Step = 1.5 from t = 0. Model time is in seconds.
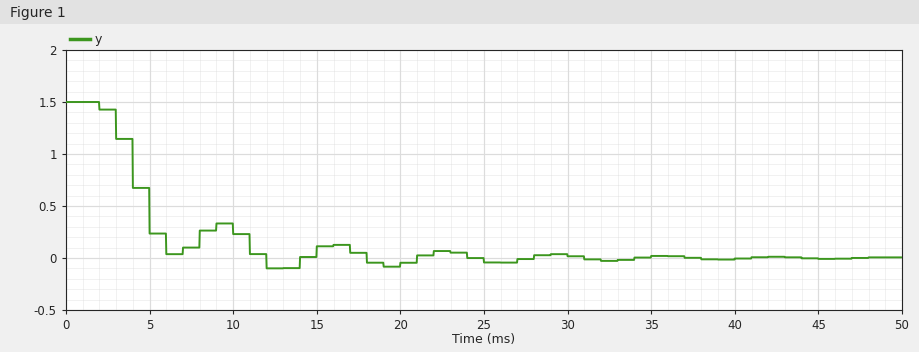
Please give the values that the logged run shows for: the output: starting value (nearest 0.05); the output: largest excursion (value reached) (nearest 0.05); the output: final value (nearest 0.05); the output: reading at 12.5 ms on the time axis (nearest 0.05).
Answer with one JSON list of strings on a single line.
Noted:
["1.50", "-0.10", "0.00", "-0.10"]
